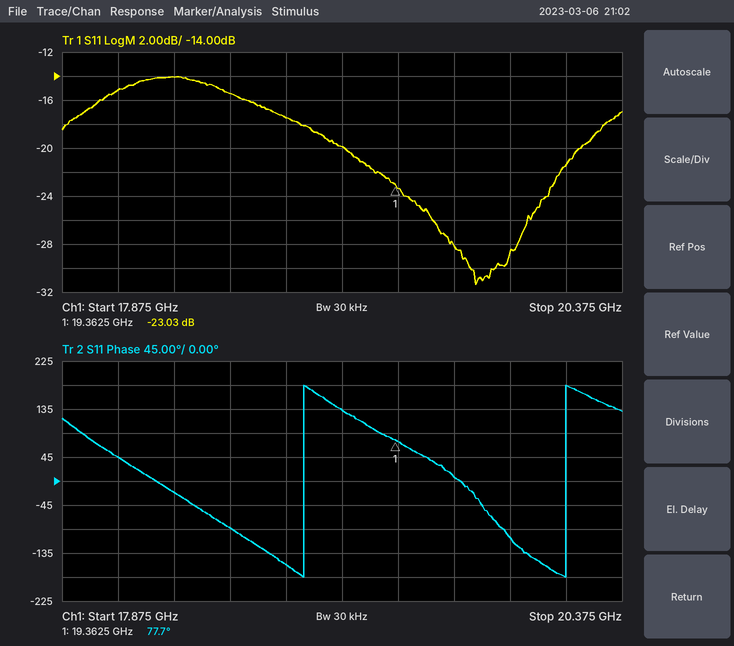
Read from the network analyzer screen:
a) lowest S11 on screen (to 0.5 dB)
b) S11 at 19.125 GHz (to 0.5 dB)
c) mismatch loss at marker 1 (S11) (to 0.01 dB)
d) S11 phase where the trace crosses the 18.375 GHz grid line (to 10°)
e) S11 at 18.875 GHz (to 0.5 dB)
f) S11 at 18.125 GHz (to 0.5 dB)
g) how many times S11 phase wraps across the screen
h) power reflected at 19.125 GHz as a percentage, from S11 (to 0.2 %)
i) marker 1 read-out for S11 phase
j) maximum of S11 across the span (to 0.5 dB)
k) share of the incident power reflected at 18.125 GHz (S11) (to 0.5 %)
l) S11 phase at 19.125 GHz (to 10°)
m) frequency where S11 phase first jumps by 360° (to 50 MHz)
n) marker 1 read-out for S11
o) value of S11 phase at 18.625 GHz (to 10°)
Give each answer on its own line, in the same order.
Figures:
-31.5 dB
-20.0 dB
0.02 dB
-20°
-17.5 dB
-15.0 dB
2
1.0 %
77.7°
-14.0 dB
3.0 %
130°
18.95 GHz
-23.03 dB
-90°
